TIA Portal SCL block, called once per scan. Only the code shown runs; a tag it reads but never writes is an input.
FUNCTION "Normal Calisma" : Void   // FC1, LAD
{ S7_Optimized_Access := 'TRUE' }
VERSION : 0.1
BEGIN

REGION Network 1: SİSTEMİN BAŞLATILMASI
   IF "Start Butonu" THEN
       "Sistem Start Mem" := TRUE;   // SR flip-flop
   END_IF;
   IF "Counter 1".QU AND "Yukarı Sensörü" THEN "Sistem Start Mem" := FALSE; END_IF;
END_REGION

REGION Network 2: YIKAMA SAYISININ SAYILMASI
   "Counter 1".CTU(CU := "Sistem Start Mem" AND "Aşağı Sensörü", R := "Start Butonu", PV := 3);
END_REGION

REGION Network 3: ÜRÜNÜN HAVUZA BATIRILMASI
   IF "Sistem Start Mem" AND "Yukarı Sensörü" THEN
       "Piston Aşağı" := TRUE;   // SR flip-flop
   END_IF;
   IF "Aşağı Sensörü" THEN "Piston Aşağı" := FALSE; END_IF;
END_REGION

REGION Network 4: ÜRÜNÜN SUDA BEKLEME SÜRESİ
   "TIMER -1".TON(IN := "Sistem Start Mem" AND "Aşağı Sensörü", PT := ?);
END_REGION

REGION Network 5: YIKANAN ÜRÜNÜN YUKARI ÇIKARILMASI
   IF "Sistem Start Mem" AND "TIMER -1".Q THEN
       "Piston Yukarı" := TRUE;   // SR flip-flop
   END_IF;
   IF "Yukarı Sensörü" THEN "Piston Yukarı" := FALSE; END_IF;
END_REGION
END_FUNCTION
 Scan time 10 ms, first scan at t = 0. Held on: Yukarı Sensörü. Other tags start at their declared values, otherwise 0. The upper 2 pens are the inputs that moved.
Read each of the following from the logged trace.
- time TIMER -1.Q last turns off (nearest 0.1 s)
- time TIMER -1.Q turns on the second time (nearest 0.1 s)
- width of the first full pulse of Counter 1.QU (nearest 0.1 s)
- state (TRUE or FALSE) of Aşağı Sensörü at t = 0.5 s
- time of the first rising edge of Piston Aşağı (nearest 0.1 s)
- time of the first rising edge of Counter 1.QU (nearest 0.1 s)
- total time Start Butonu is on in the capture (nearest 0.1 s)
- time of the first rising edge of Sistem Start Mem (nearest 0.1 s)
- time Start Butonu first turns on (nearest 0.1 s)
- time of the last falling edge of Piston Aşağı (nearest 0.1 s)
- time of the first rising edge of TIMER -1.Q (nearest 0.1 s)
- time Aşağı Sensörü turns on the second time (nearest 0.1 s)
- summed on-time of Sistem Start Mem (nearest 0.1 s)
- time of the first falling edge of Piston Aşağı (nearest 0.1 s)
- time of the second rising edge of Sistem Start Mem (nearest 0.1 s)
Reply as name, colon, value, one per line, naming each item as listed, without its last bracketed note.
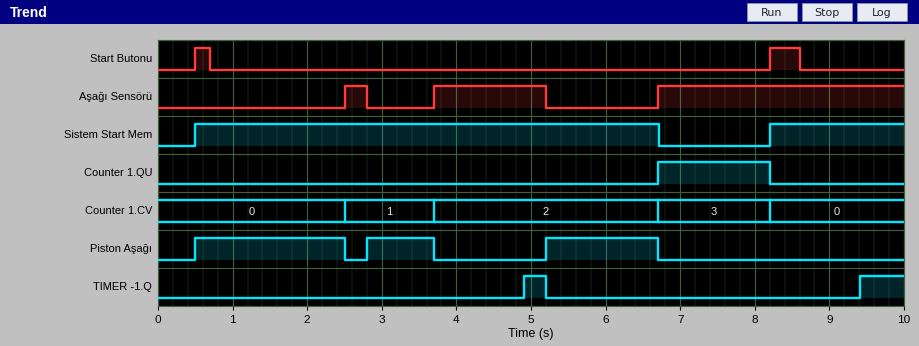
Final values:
time TIMER -1.Q last turns off: 5.2 s
time TIMER -1.Q turns on the second time: 9.4 s
width of the first full pulse of Counter 1.QU: 1.5 s
state (TRUE or FALSE) of Aşağı Sensörü at t = 0.5 s: FALSE
time of the first rising edge of Piston Aşağı: 0.5 s
time of the first rising edge of Counter 1.QU: 6.7 s
total time Start Butonu is on in the capture: 0.6 s
time of the first rising edge of Sistem Start Mem: 0.5 s
time Start Butonu first turns on: 0.5 s
time of the last falling edge of Piston Aşağı: 6.7 s
time of the first rising edge of TIMER -1.Q: 4.9 s
time Aşağı Sensörü turns on the second time: 3.7 s
summed on-time of Sistem Start Mem: 8.0 s
time of the first falling edge of Piston Aşağı: 2.5 s
time of the second rising edge of Sistem Start Mem: 8.2 s
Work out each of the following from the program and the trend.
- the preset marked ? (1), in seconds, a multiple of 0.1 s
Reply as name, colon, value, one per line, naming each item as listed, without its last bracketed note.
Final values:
the preset marked ? (1), in seconds, a multiple of 0.1 s: 1.2 s
